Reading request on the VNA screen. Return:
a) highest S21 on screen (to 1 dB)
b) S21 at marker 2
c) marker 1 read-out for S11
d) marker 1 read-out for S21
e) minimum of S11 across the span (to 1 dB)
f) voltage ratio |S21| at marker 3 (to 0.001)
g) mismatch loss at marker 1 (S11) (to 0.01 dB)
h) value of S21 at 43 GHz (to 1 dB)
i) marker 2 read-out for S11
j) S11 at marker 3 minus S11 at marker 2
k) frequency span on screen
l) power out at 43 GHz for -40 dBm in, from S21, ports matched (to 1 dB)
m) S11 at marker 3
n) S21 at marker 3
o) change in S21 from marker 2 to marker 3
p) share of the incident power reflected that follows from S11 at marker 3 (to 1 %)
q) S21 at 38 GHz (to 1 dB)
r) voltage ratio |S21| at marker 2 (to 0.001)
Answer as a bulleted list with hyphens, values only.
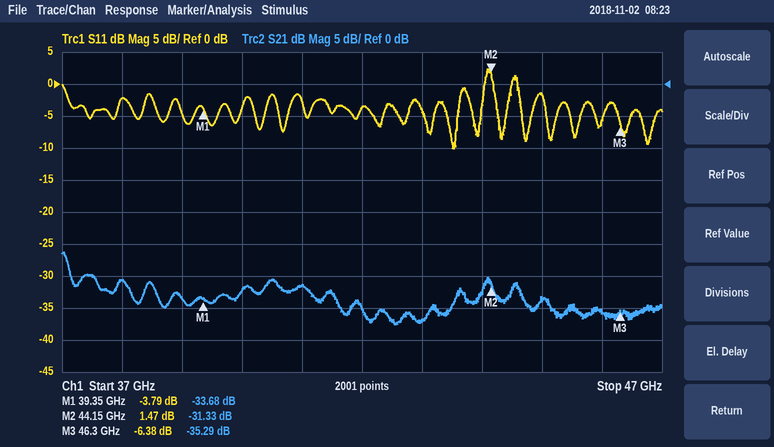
- -26 dB
- -31.33 dB
- -3.79 dB
- -33.68 dB
- -10 dB
- 0.017
- 2.35 dB
- -37 dB
- 1.47 dB
- -7.85 dB
- 10 GHz
- -77 dBm
- -6.38 dB
- -35.29 dB
- -3.96 dB
- 23 %
- -31 dB
- 0.027
